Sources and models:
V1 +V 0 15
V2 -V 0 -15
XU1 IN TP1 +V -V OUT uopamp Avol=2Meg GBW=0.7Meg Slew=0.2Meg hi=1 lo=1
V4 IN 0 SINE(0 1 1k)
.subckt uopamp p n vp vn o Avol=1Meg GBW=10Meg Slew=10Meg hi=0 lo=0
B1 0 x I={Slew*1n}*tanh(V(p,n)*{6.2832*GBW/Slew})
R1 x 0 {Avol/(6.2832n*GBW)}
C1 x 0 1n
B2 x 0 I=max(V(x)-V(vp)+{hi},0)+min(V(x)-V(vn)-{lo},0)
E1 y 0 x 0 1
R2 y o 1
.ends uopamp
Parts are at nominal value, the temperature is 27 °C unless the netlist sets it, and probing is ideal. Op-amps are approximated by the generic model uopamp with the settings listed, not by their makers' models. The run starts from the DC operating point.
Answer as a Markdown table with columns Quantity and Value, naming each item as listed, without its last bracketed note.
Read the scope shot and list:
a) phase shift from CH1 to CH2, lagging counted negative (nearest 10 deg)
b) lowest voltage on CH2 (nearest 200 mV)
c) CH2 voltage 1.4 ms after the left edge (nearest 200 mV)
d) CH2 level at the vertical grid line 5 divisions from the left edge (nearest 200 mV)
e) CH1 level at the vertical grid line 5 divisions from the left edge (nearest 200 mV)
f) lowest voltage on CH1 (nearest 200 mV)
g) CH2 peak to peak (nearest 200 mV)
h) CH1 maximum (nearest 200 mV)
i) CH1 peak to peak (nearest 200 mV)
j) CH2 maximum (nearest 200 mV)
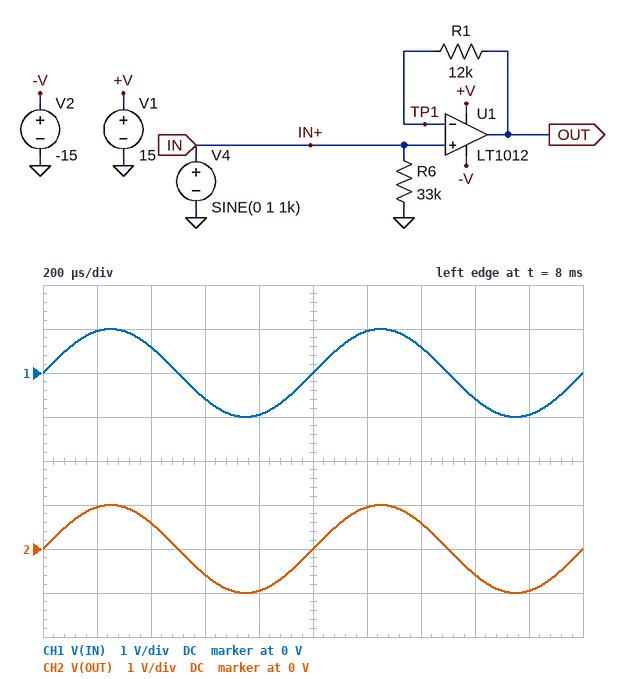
| Quantity | Value |
|---|---|
| phase shift from CH1 to CH2, lagging counted negative | 0 deg |
| lowest voltage on CH2 | -1.0 V |
| CH2 voltage 1.4 ms after the left edge | 600 mV |
| CH2 level at the vertical grid line 5 divisions from the left edge | 0 V |
| CH1 level at the vertical grid line 5 divisions from the left edge | 0 V |
| lowest voltage on CH1 | -1.0 V |
| CH2 peak to peak | 2.0 V |
| CH1 maximum | 1.0 V |
| CH1 peak to peak | 2.0 V |
| CH2 maximum | 1.0 V |
